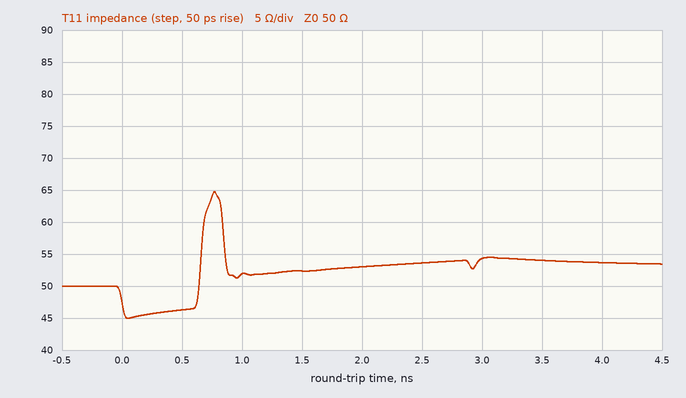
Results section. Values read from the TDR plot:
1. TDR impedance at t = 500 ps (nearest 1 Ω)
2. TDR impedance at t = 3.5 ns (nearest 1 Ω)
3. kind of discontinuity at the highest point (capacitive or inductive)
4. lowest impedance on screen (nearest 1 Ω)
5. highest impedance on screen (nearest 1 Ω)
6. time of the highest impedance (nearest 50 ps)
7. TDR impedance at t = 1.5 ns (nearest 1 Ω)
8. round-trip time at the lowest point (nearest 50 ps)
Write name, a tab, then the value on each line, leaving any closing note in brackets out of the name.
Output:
TDR impedance at t = 500 ps	46 Ω
TDR impedance at t = 3.5 ns	54 Ω
kind of discontinuity at the highest point	inductive
lowest impedance on screen	45 Ω
highest impedance on screen	65 Ω
time of the highest impedance	750 ps
TDR impedance at t = 1.5 ns	52 Ω
round-trip time at the lowest point	50 ps
